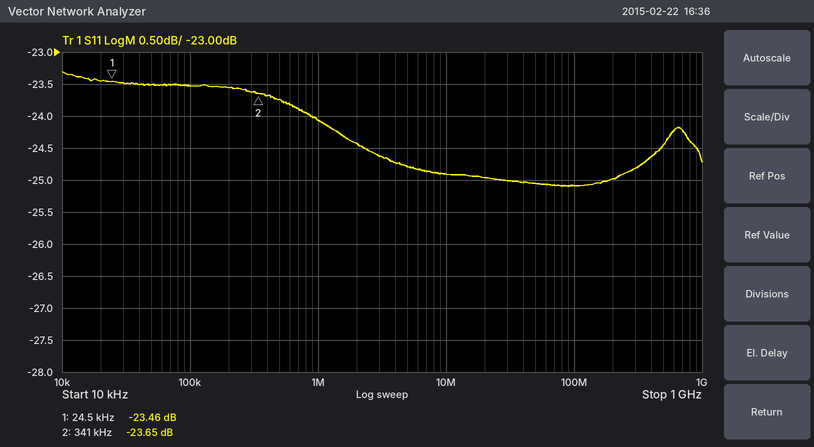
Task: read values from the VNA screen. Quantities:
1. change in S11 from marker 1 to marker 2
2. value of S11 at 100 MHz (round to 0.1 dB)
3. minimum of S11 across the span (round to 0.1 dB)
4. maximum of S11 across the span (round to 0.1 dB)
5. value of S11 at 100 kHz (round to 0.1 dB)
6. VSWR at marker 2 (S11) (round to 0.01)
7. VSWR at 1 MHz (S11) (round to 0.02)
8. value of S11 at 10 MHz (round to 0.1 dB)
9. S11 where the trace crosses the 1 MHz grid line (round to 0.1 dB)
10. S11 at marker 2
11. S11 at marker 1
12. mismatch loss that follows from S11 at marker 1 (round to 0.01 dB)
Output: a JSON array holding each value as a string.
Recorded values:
["-0.19 dB", "-25.1 dB", "-25.1 dB", "-23.3 dB", "-23.5 dB", "1.14", "1.14", "-24.9 dB", "-24.1 dB", "-23.65 dB", "-23.46 dB", "0.02 dB"]
